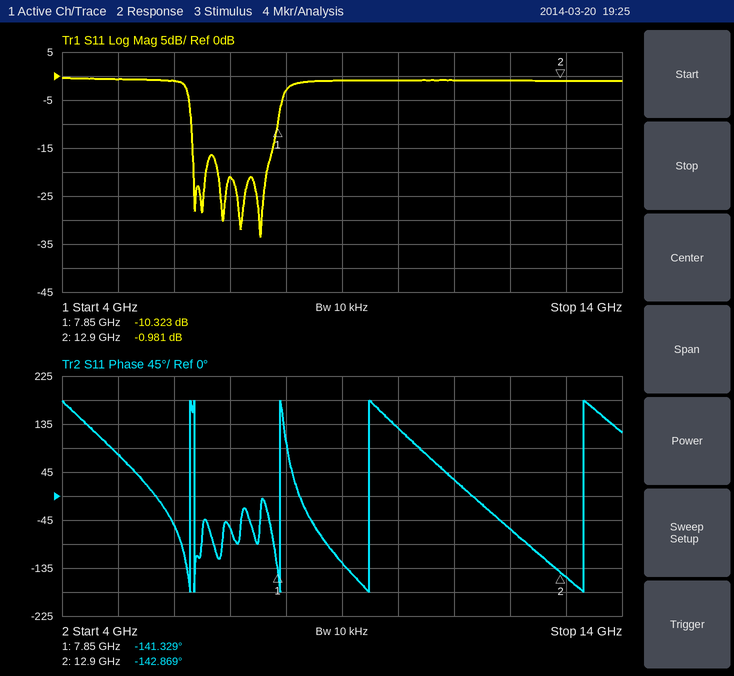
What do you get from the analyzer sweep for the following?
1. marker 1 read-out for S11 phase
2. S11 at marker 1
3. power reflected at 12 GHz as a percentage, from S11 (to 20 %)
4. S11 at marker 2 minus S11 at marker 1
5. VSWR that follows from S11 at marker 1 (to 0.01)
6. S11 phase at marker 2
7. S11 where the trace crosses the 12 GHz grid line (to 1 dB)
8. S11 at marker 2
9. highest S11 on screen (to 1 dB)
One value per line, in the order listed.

-141.329°
-10.323 dB
80 %
9.342 dB
1.88
-142.869°
-1 dB
-0.981 dB
0 dB
